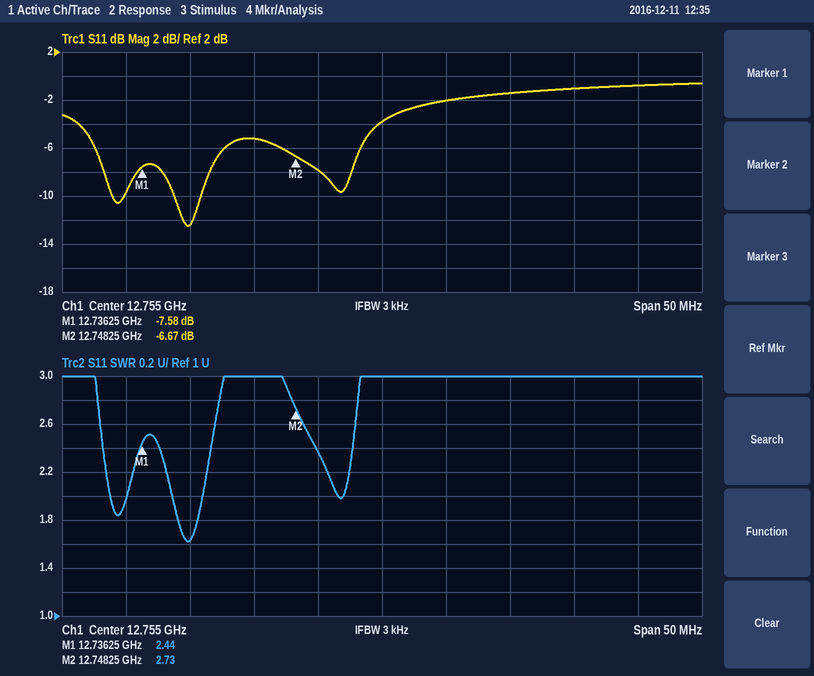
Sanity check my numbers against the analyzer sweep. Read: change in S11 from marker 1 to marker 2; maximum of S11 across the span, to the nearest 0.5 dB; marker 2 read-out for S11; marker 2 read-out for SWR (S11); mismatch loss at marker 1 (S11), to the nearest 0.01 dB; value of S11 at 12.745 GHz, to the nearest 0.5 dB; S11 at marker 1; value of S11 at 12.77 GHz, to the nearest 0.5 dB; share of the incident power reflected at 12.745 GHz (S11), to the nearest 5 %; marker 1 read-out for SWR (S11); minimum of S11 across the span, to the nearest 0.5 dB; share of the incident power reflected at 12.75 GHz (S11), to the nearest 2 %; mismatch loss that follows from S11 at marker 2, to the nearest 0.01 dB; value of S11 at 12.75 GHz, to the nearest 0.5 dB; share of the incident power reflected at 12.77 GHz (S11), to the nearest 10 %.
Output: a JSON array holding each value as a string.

["0.91 dB", "-0.5 dB", "-6.67 dB", "2.73", "0.83 dB", "-5.0 dB", "-7.58 dB", "-1.0 dB", "30 %", "2.44", "-12.5 dB", "16 %", "1.05 dB", "-8.0 dB", "80 %"]
